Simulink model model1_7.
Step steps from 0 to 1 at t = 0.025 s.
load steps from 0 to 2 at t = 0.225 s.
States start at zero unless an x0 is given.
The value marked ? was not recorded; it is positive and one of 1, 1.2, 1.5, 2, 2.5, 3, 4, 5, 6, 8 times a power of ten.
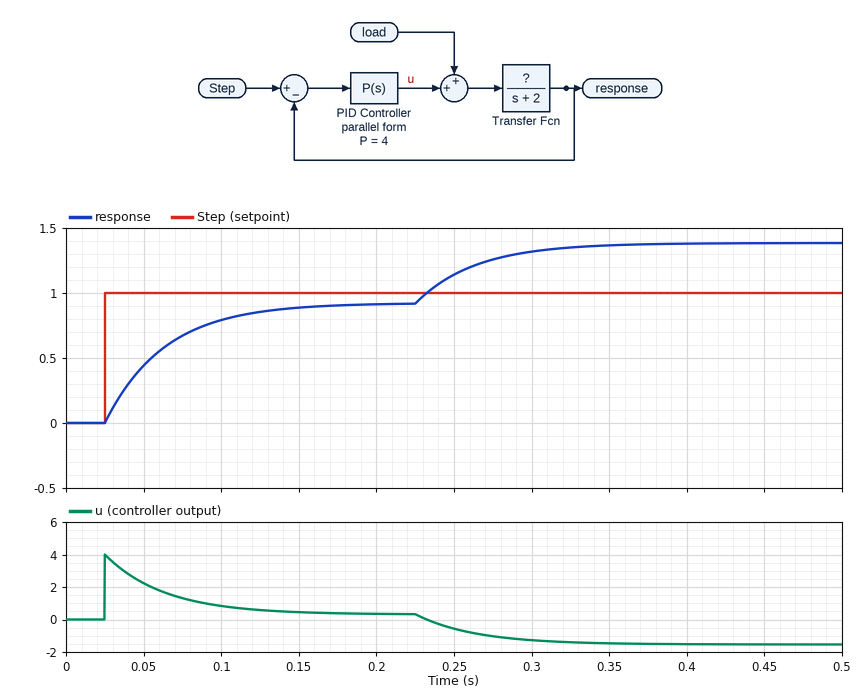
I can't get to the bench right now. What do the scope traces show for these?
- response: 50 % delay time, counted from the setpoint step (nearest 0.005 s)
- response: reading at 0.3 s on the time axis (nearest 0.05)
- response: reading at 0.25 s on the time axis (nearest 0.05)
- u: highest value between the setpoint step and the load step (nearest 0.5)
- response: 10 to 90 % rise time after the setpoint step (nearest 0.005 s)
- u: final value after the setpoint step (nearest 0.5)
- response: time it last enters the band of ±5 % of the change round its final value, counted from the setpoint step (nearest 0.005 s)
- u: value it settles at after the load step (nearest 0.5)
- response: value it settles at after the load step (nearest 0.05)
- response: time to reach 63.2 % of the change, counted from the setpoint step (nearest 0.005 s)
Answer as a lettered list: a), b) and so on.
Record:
a) 0.025 s
b) 1.30
c) 1.15
d) 4.0
e) 0.085 s
f) 0.5
g) 0.115 s
h) -1.5
i) 1.40
j) 0.040 s
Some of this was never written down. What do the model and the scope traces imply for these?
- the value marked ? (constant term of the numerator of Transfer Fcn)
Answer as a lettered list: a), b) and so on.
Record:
a) 6
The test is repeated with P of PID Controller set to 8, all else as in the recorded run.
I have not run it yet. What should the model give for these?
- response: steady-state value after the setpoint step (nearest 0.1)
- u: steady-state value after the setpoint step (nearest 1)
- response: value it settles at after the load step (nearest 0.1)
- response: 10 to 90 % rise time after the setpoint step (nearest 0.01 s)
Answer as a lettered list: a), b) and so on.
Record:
a) 1.0
b) 0
c) 1.2
d) 0.04 s
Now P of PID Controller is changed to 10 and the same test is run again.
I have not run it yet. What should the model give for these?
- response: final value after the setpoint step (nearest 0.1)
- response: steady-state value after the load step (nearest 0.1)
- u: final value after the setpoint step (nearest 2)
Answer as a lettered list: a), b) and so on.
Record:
a) 1.0
b) 1.2
c) 0
